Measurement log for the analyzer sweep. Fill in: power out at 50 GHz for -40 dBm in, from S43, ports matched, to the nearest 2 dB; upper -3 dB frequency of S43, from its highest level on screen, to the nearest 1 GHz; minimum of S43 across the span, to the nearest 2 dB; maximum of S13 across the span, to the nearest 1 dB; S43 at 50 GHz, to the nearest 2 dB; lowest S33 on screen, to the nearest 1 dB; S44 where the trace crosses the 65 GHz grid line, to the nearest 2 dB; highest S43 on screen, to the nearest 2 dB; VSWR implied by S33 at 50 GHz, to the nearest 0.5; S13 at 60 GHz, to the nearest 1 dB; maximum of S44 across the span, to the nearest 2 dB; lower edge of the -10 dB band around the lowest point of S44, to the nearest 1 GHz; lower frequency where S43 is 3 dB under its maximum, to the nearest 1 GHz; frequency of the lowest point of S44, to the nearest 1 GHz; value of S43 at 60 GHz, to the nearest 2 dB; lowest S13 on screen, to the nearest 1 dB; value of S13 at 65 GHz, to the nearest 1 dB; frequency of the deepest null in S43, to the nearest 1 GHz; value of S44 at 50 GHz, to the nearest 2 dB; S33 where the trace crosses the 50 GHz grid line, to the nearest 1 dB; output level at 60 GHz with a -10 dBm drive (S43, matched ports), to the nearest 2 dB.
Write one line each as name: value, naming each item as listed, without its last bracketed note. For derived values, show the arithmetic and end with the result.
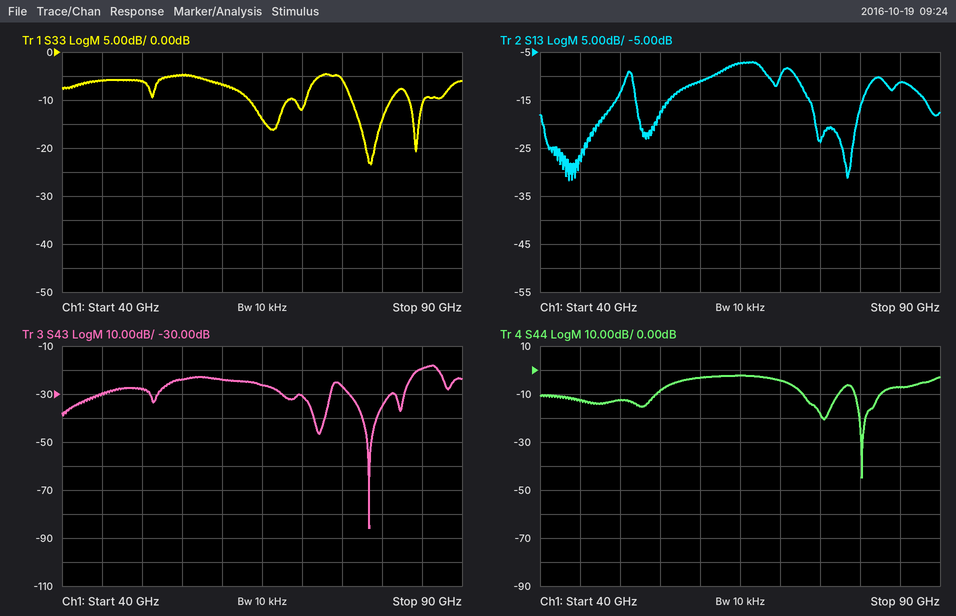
power out at 50 GHz for -40 dBm in, from S43, ports matched, to the nearest 2 dB: -40 dBm + (-28 dB) = -68 dBm
upper -3 dB frequency of S43, from its highest level on screen, to the nearest 1 GHz: 87 GHz
minimum of S43 across the span, to the nearest 2 dB: -86 dB
maximum of S13 across the span, to the nearest 1 dB: -7 dB
S43 at 50 GHz, to the nearest 2 dB: -28 dB
lowest S33 on screen, to the nearest 1 dB: -23 dB
S44 where the trace crosses the 65 GHz grid line, to the nearest 2 dB: -2 dB
highest S43 on screen, to the nearest 2 dB: -18 dB
VSWR implied by S33 at 50 GHz, to the nearest 0.5: |Γ| = 10^(-6/20) = 0.5012; VSWR = (1 + 0.5012)/(1 − 0.5012) ≈ 3.0
S13 at 60 GHz, to the nearest 1 dB: -11 dB
maximum of S44 across the span, to the nearest 2 dB: -2 dB
lower edge of the -10 dB band around the lowest point of S44, to the nearest 1 GHz: 79 GHz
lower frequency where S43 is 3 dB under its maximum, to the nearest 1 GHz: 84 GHz
frequency of the lowest point of S44, to the nearest 1 GHz: 80 GHz
value of S43 at 60 GHz, to the nearest 2 dB: -24 dB
lowest S13 on screen, to the nearest 1 dB: -32 dB
value of S13 at 65 GHz, to the nearest 1 dB: -7 dB
frequency of the deepest null in S43, to the nearest 1 GHz: 78 GHz
value of S44 at 50 GHz, to the nearest 2 dB: -12 dB
S33 where the trace crosses the 50 GHz grid line, to the nearest 1 dB: -6 dB
output level at 60 GHz with a -10 dBm drive (S43, matched ports), to the nearest 2 dB: -10 dBm + (-24 dB) = -34 dBm
